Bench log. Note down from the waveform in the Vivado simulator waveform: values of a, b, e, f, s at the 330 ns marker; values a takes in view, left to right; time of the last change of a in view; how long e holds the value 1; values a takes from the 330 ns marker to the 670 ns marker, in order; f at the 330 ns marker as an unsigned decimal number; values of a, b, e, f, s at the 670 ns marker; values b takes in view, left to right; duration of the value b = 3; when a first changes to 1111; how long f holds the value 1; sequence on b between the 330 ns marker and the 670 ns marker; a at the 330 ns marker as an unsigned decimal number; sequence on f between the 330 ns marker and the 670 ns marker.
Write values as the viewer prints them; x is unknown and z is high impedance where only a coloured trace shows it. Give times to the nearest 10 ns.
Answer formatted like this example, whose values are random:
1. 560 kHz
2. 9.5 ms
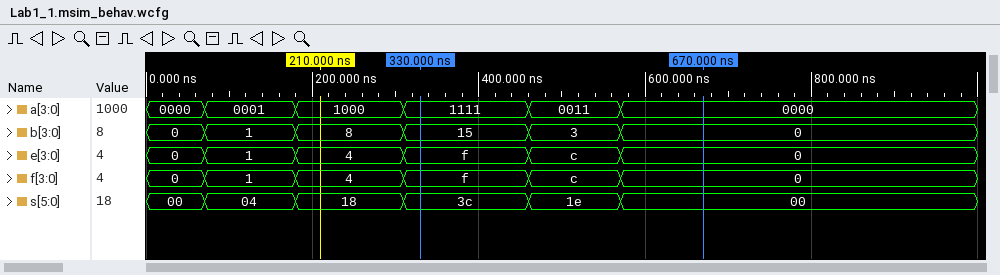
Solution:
1. a=1111, b=15, e=f, f=f, s=3c
2. 0000, 0001, 1000, 1111, 0011, 0000
3. 570 ns
4. 110 ns
5. 1111, 0011, 0000
6. 15
7. a=0000, b=0, e=0, f=0, s=00
8. 0, 1, 8, 15, 3, 0
9. 110 ns
10. 310 ns
11. 110 ns
12. 15, 3, 0
13. 15
14. f, c, 0
